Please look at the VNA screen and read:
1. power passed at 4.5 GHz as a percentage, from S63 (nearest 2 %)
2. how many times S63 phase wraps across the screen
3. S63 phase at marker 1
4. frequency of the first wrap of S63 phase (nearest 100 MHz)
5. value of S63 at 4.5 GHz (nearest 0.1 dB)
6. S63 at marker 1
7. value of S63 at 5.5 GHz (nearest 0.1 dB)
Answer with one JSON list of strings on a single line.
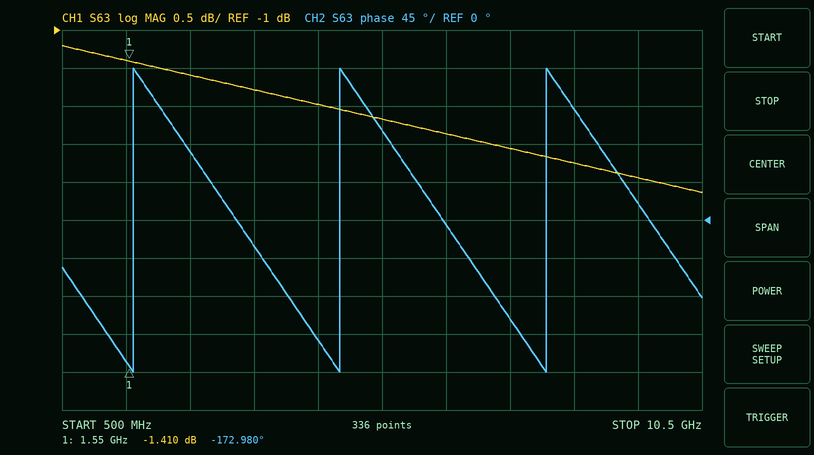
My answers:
["64 %", "3", "-172.980°", "1.6 GHz", "-2.0 dB", "-1.410 dB", "-2.2 dB"]
